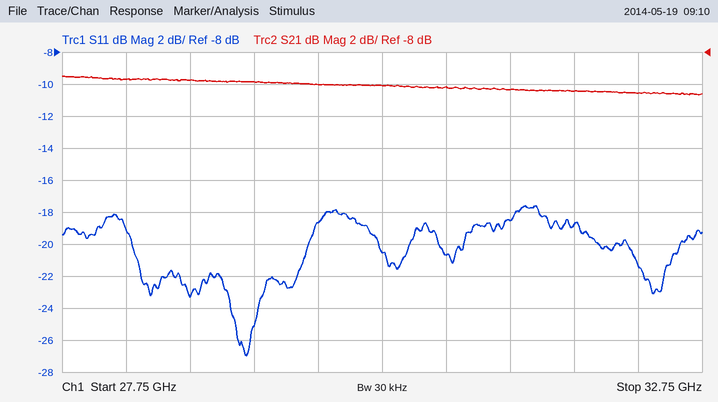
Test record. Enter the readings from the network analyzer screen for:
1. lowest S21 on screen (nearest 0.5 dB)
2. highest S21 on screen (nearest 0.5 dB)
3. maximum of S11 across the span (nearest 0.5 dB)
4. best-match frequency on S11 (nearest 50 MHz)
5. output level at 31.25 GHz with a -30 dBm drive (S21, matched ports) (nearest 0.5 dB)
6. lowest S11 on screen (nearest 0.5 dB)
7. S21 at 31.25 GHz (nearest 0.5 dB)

-10.5 dB
-9.5 dB
-17.5 dB
29.20 GHz
-40.5 dBm
-27.0 dB
-10.5 dB
